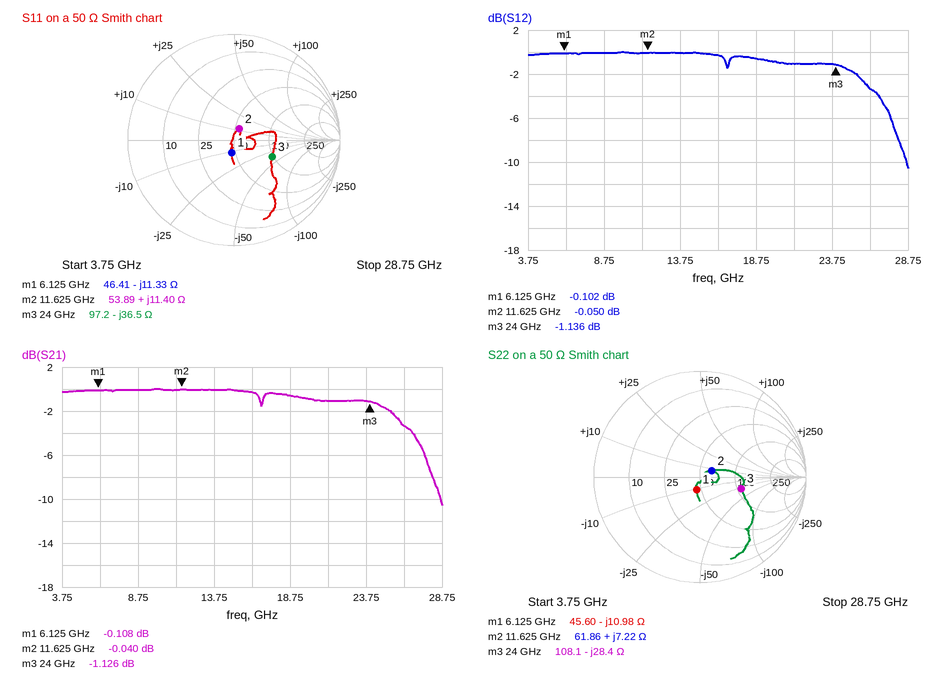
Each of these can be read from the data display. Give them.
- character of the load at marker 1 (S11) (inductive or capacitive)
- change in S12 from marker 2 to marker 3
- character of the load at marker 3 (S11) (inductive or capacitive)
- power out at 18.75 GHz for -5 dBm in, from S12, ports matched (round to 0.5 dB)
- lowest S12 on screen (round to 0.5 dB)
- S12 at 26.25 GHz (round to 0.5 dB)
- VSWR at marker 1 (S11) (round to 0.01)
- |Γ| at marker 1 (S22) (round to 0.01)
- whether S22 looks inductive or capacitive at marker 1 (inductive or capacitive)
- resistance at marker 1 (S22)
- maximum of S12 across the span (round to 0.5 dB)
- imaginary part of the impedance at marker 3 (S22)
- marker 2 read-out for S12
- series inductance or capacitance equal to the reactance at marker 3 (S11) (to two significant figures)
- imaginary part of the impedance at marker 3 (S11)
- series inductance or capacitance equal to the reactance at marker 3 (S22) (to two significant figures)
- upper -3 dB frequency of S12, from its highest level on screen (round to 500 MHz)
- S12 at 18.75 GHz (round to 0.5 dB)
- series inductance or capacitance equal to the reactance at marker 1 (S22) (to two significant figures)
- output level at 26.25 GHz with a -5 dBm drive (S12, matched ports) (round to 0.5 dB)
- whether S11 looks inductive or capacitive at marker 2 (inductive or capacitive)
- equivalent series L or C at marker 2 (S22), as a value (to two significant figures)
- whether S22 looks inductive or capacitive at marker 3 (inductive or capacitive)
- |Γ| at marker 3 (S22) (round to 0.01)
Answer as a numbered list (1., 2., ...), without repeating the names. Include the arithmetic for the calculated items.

1. capacitive
2. -1.136 − (-0.05) = -1.086 dB
3. capacitive
4. -5 dBm + (-0.5 dB) = -5.5 dBm
5. -10.5 dB
6. -3.5 dB
7. 1.28
8. 0.12
9. capacitive
10. 45.60 Ω
11. 0.0 dB
12. -28.4 Ω
13. -0.050 dB
14. C = 1/(2π × 24 GHz × 36.5 Ω) ≈ 182 fF, so 180 fF to two significant figures
15. -36.5 Ω
16. C = 1/(2π × 24 GHz × 28.4 Ω) ≈ 234 fF, so 230 fF to two significant figures
17. 26.0 GHz
18. -0.5 dB
19. C = 1/(2π × 6.125 GHz × 10.98 Ω) ≈ 2.4 pF
20. -5 dBm + (-3.5 dB) = -8.5 dBm
21. inductive
22. L = 7.22 Ω/(2π × 11.625 GHz) ≈ 99 pH
23. capacitive
24. 0.40
